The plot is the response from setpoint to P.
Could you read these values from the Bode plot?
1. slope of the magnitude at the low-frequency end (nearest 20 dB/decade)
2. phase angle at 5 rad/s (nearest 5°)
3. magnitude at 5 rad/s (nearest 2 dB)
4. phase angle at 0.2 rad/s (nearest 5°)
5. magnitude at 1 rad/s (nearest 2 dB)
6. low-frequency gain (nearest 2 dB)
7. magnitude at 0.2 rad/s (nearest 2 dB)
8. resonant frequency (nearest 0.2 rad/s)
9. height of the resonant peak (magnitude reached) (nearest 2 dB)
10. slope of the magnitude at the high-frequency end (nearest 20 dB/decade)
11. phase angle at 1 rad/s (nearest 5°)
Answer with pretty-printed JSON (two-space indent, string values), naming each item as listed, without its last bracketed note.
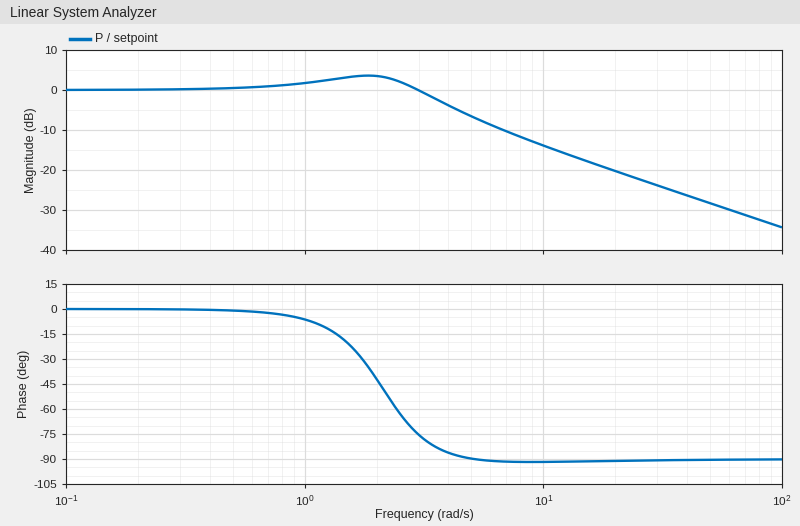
{
  "slope of the magnitude at the low-frequency end": "0 dB/decade",
  "phase angle at 5 rad/s": "-90°",
  "magnitude at 5 rad/s": "-6 dB",
  "phase angle at 0.2 rad/s": "0°",
  "magnitude at 1 rad/s": "2 dB",
  "low-frequency gain": "0 dB",
  "magnitude at 0.2 rad/s": "0 dB",
  "resonant frequency": "1.8 rad/s",
  "height of the resonant peak (magnitude reached)": "4 dB",
  "slope of the magnitude at the high-frequency end": "-20 dB/decade",
  "phase angle at 1 rad/s": "-5°"
}
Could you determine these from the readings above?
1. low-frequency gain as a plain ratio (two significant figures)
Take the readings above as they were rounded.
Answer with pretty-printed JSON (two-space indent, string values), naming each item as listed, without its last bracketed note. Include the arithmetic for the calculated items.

{
  "low-frequency gain as a plain ratio": "10^(0 / 20) = 1.0"
}
